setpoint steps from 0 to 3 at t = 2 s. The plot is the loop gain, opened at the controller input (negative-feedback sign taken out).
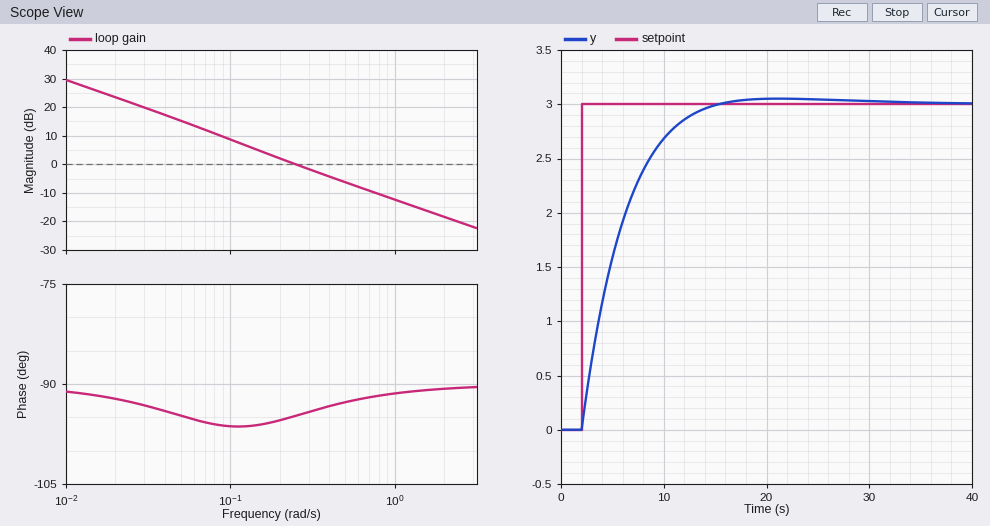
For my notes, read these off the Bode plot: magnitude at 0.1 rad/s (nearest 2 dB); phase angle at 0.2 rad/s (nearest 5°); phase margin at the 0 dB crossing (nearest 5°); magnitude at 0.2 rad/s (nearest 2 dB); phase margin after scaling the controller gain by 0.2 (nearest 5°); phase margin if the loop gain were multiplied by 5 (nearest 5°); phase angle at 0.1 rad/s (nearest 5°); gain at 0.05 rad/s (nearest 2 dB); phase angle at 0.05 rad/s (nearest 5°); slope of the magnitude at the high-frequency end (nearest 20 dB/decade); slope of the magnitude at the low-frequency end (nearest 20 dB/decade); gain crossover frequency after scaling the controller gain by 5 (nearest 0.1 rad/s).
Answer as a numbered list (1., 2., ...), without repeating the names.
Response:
1. 8 dB
2. -95°
3. 85°
4. 2 dB
5. 85°
6. 90°
7. -95°
8. 16 dB
9. -95°
10. -20 dB/decade
11. -20 dB/decade
12. 1.2 rad/s
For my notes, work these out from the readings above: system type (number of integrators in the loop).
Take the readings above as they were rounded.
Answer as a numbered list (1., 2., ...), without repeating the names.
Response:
1. 1
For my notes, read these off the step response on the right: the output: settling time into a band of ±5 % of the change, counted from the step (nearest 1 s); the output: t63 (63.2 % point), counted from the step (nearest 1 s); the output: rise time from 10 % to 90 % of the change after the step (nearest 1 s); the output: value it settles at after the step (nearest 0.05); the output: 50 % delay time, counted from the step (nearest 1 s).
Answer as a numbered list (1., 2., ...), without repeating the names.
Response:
1. 10 s
2. 4 s
3. 8 s
4. 3.00
5. 3 s
